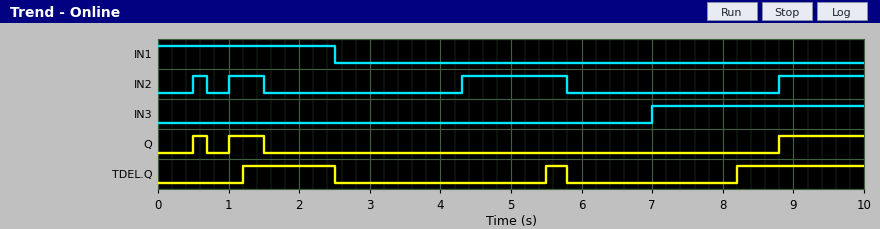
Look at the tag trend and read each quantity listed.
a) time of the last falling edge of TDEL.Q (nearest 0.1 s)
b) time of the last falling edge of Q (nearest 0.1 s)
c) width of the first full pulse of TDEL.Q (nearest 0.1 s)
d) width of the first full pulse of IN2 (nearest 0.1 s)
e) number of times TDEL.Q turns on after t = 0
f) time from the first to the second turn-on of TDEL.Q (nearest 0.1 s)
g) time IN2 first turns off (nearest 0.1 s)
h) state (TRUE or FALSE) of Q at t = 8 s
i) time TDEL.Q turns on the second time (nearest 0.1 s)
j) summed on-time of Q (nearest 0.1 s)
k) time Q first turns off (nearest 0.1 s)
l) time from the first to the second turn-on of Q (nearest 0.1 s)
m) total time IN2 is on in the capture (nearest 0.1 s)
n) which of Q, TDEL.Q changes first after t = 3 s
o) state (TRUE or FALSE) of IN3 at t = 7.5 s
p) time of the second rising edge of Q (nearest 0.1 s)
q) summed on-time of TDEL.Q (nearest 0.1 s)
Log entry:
5.8 s
1.5 s
1.3 s
0.2 s
3
4.3 s
0.7 s
FALSE
5.5 s
1.9 s
0.7 s
0.5 s
3.4 s
TDEL.Q
TRUE
1.0 s
3.4 s
